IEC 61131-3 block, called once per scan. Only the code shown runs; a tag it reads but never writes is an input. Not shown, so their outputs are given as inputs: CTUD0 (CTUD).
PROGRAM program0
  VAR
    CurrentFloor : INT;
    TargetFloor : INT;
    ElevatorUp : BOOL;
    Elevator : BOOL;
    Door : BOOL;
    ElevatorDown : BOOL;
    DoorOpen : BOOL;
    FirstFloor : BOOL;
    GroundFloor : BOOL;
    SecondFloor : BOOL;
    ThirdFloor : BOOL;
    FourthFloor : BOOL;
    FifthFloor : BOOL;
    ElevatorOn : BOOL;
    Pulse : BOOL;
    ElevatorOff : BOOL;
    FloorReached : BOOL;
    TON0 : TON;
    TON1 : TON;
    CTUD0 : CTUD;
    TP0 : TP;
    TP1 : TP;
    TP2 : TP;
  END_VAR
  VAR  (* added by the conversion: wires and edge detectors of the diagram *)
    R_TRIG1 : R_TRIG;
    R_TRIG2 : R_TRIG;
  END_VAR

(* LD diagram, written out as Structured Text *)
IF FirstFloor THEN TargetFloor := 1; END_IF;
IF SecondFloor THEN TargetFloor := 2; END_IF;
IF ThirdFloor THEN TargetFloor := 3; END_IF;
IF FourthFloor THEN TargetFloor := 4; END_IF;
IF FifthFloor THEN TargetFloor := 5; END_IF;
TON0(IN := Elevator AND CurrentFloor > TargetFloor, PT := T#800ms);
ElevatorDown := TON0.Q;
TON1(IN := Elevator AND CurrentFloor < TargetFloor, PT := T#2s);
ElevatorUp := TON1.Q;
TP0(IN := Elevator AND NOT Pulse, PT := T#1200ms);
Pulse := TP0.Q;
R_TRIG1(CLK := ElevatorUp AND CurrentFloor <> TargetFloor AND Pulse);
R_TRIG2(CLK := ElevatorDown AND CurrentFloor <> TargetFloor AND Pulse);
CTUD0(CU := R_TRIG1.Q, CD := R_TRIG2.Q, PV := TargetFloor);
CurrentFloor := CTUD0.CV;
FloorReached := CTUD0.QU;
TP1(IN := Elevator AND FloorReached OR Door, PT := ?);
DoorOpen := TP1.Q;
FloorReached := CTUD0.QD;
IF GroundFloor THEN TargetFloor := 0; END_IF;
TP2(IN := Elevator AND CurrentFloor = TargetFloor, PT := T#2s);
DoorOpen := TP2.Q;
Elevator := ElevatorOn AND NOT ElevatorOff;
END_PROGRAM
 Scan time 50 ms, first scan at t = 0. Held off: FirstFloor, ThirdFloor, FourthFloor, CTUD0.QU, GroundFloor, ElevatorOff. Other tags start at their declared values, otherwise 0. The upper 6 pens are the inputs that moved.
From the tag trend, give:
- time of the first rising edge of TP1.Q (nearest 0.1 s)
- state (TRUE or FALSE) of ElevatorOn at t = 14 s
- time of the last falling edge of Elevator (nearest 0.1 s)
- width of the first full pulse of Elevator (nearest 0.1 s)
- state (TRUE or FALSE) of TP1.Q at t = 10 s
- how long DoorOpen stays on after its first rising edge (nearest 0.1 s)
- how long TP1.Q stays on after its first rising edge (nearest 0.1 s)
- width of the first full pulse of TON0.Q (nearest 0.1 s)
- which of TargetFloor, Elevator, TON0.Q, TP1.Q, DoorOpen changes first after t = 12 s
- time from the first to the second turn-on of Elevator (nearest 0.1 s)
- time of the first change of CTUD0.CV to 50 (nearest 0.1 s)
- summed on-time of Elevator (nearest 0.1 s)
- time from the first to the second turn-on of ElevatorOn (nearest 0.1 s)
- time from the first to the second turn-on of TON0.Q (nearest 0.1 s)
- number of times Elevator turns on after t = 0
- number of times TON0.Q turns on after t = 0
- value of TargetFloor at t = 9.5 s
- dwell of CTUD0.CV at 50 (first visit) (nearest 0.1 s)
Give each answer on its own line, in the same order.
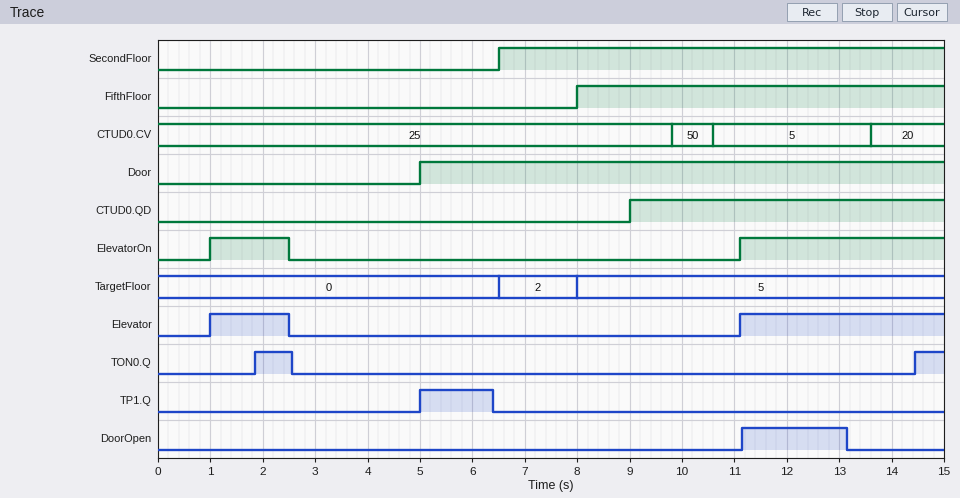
5.0 s
TRUE
2.5 s
1.5 s
FALSE
2.0 s
1.4 s
0.7 s
DoorOpen
10.1 s
9.8 s
5.4 s
10.1 s
12.6 s
2
2
5
0.8 s
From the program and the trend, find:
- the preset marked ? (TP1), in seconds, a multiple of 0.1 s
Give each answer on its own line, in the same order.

1.4 s
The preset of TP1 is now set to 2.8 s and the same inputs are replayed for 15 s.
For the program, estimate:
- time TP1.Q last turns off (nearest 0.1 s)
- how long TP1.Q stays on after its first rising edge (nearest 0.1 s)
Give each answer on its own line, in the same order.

7.8 s
2.8 s
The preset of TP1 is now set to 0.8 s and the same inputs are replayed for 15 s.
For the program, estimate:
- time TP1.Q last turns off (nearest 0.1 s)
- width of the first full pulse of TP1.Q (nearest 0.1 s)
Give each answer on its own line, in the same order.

5.8 s
0.8 s
